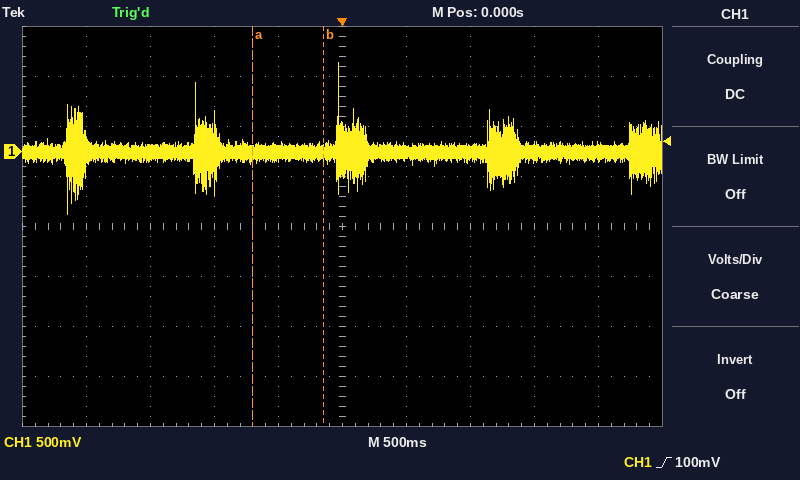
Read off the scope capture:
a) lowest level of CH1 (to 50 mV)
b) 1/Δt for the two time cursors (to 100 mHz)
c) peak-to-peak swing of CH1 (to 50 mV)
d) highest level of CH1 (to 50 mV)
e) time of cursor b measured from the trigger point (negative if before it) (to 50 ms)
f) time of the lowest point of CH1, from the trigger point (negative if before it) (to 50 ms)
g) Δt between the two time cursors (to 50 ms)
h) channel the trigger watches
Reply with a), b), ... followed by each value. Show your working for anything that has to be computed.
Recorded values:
a) -600 mV
b) 1 / 550 ms ≈ 1.8 Hz
c) 900 mV − (-600 mV) = 1.50 V
d) 900 mV
e) -150 ms
f) -2.15 s
g) 550 ms
h) CH1
